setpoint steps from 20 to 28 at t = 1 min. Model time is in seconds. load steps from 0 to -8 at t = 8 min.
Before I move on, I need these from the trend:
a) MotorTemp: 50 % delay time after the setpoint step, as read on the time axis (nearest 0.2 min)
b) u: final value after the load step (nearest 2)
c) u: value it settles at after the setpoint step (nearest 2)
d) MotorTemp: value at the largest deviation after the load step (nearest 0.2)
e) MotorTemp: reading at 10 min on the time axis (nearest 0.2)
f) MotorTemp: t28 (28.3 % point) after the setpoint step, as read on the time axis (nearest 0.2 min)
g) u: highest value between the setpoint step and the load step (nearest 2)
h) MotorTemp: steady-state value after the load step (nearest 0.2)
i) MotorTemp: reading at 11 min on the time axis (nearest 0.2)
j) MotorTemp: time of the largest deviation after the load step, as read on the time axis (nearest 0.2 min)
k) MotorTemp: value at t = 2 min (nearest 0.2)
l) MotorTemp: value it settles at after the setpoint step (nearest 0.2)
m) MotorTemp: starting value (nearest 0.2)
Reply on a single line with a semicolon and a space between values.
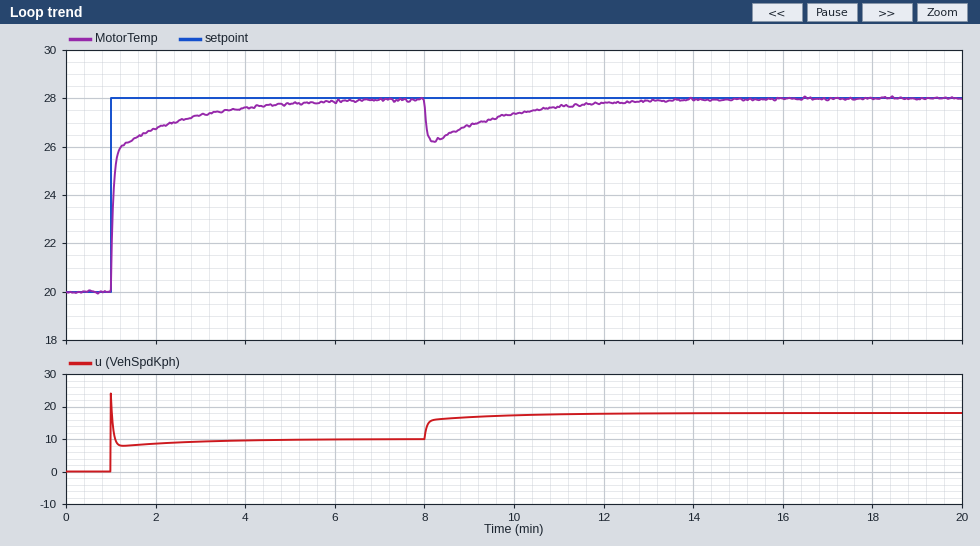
1.0 min; 18; 10; 26.2; 27.4; 1.0 min; 24; 28.0; 27.6; 8.2 min; 26.8; 28.0; 20.0
